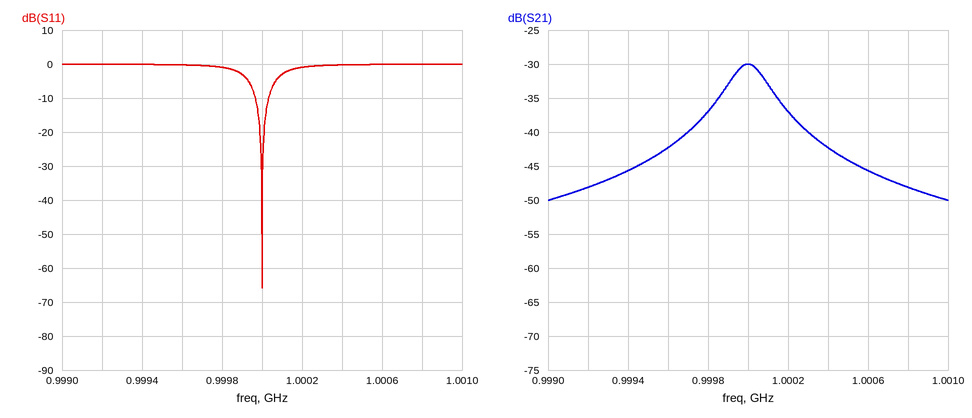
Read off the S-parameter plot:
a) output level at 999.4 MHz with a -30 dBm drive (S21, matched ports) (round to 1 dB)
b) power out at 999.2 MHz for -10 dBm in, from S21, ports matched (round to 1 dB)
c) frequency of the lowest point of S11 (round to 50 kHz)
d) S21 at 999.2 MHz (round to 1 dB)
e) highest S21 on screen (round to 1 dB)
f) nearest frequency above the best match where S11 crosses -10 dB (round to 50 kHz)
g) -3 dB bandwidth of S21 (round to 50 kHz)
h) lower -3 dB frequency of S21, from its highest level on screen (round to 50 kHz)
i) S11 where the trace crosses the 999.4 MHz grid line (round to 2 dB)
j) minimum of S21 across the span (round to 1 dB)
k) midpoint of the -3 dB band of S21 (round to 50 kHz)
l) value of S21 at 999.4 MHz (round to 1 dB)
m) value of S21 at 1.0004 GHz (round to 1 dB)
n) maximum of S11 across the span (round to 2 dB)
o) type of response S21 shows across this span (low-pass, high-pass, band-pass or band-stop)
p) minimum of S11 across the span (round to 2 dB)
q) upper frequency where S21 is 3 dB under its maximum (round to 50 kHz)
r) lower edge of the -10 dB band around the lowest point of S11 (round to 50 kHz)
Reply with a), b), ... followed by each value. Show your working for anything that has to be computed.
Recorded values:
a) -30 dBm + (-46 dB) = -76 dBm
b) -10 dBm + (-48 dB) = -58 dBm
c) 1.00000 GHz
d) -48 dB
e) -30 dB
f) 1.00005 GHz
g) 1.00010 GHz − 999.90 MHz = 200 kHz
h) 999.90 MHz
i) 0 dB
j) -50 dB
k) 1.00000 GHz
l) -46 dB
m) -42 dB
n) 0 dB
o) band-pass
p) -66 dB
q) 1.00010 GHz
r) 999.95 MHz
